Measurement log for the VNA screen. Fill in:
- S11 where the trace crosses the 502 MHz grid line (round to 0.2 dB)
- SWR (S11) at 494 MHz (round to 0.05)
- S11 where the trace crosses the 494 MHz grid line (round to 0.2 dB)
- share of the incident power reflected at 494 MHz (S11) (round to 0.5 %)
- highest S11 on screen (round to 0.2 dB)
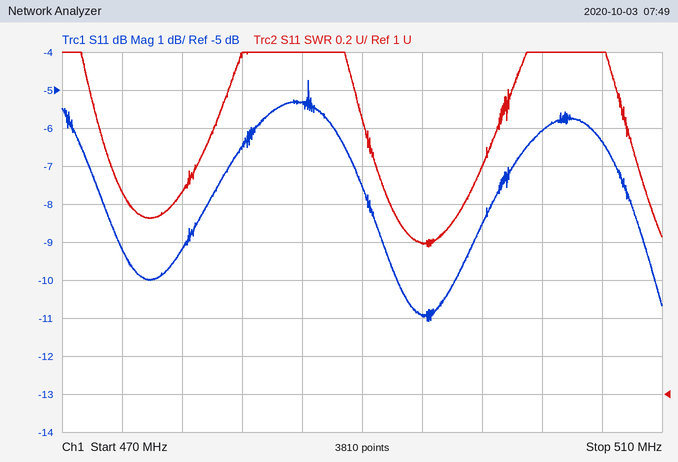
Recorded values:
-6.0 dB
1.80
-11.0 dB
8.0 %
-4.8 dB
